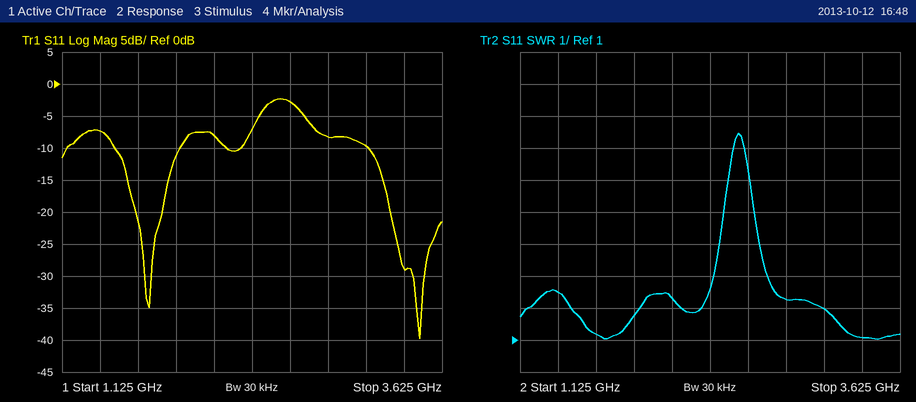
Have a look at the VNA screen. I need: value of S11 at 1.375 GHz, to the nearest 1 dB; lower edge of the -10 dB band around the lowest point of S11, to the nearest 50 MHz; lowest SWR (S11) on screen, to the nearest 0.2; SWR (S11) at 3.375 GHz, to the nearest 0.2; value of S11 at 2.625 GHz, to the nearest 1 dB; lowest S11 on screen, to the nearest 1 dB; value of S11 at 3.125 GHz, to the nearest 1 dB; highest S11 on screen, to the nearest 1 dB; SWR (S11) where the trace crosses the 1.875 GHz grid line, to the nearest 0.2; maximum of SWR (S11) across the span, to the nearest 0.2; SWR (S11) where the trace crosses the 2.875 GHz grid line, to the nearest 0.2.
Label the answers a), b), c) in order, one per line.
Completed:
a) -7 dB
b) 3.15 GHz
c) 1.0
d) 1.0
e) -3 dB
f) -40 dB
g) -10 dB
h) -2 dB
i) 1.8
j) 7.4
k) 2.2
